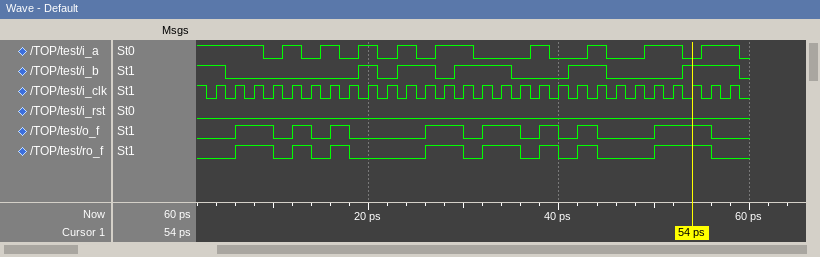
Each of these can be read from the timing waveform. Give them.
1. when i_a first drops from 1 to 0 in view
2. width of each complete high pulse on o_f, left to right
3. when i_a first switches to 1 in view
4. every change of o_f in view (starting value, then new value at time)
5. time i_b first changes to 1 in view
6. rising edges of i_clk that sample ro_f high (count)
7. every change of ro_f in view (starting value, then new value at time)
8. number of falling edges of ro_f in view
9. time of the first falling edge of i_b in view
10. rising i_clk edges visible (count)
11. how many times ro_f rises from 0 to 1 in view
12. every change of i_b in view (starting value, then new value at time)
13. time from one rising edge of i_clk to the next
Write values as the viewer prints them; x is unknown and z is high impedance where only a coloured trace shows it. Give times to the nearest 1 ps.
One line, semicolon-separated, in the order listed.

9 ps; 4 ps, 2 ps, 2 ps, 4 ps, 4 ps, 2 ps, 2 ps, 6 ps; 11 ps; 0, 1 at 6 ps, 0 at 10 ps, 1 at 12 ps, 0 at 14 ps, 1 at 16 ps, 0 at 18 ps, 1 at 26 ps, 0 at 30 ps, 1 at 32 ps, 0 at 36 ps, 1 at 38 ps, 0 at 40 ps, 1 at 42 ps, 0 at 44 ps, 1 at 50 ps, 0 at 56 ps; 19 ps; 13; 0, 1 at 6 ps, 0 at 10 ps, 1 at 12 ps, 0 at 14 ps, 1 at 16 ps, 0 at 18 ps, 1 at 26 ps, 0 at 30 ps, 1 at 32 ps, 0 at 36 ps, 1 at 38 ps, 0 at 40 ps, 1 at 42 ps, 0 at 44 ps, 1 at 50 ps, 0 at 56 ps; 8; 5 ps; 28; 8; 1, 0 at 5 ps, 1 at 19 ps, 0 at 21 ps, 1 at 23 ps, 0 at 27 ps, 1 at 29 ps, 0 at 35 ps, 1 at 41 ps, 0 at 45 ps, 1 at 53 ps, 0 at 59 ps; 2 ps
